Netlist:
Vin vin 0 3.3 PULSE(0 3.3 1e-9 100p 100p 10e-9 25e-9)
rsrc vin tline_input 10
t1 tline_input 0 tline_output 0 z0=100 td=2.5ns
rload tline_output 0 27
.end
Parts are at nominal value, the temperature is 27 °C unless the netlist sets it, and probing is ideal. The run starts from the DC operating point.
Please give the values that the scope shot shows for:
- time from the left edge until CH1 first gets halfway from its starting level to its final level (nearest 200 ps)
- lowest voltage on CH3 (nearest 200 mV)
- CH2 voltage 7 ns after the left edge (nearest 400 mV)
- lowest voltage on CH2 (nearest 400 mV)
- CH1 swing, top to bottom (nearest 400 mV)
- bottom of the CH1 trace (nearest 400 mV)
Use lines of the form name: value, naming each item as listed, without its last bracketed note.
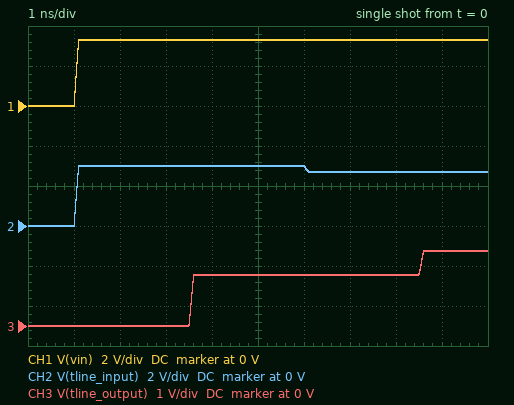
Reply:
time from the left edge until CH1 first gets halfway from its starting level to its final level: 1.0 ns
lowest voltage on CH3: 0 V
CH2 voltage 7 ns after the left edge: 2.8 V
lowest voltage on CH2: 0 V
CH1 swing, top to bottom: 3.2 V
bottom of the CH1 trace: 0 V
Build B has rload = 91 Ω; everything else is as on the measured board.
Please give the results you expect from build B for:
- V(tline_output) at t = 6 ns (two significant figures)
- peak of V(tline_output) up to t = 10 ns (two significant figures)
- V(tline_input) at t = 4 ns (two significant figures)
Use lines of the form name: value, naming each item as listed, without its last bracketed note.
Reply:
V(tline_output) at t = 6 ns: 2.9 V
peak of V(tline_output) up to t = 10 ns: 3.0 V
V(tline_input) at t = 4 ns: 3.0 V
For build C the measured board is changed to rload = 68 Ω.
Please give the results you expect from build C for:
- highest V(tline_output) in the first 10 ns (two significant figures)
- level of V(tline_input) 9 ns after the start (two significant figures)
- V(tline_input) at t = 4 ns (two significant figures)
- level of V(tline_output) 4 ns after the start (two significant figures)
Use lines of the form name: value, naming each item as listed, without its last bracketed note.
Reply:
highest V(tline_output) in the first 10 ns: 2.8 V
level of V(tline_input) 9 ns after the start: 2.9 V
V(tline_input) at t = 4 ns: 3.0 V
level of V(tline_output) 4 ns after the start: 2.4 V
